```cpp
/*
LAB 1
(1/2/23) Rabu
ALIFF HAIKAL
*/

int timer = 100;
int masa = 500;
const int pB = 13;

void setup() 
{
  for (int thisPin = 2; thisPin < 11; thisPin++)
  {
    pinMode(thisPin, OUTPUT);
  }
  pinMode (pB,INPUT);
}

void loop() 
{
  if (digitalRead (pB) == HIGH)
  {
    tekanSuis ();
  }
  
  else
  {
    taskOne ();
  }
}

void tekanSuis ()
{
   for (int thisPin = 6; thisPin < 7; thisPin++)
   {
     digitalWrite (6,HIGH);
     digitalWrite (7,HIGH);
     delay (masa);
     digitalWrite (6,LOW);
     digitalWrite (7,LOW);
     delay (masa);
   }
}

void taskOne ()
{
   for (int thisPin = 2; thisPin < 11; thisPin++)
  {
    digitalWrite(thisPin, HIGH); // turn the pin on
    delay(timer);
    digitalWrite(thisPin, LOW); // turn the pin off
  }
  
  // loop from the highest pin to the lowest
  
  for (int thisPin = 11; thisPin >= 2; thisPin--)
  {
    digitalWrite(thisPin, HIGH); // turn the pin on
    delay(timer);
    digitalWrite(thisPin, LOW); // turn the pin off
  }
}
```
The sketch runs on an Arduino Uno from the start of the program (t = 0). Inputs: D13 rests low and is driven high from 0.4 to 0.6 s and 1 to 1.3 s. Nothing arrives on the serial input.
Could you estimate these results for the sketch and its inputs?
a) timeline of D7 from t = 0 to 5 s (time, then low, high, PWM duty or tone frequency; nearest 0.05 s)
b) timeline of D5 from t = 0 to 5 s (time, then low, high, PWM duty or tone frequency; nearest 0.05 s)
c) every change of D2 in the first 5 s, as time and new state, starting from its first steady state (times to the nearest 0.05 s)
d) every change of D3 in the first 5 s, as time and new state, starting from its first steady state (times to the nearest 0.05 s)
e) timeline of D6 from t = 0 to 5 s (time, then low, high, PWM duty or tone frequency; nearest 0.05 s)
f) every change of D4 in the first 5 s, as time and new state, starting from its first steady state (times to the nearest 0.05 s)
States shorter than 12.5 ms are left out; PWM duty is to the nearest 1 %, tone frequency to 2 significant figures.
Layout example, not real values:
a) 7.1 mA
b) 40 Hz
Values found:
a) 0 s low; 0.5 s high; 0.6 s low; 1.3 s high; 1.4 s low; 2.4 s high; 2.5 s low; 3.2 s high; 3.3 s low; 4.3 s high; 4.4 s low
b) 0 s low; 0.3 s high; 0.4 s low; 1.5 s high; 1.6 s low; 2.2 s high; 2.3 s low; 3.4 s high; 3.5 s low; 4.1 s high; 4.2 s low
c) 0 s high; 0.1 s low; 1.8 s high; 2 s low; 3.7 s high; 3.9 s low
d) 0 s low; 0.1 s high; 0.2 s low; 1.7 s high; 1.8 s low; 2 s high; 2.1 s low; 3.6 s high; 3.7 s low; 3.9 s high; 4 s low
e) 0 s low; 0.4 s high; 0.5 s low; 1.4 s high; 1.5 s low; 2.3 s high; 2.4 s low; 3.3 s high; 3.4 s low; 4.2 s high; 4.3 s low
f) 0 s low; 0.2 s high; 0.3 s low; 1.6 s high; 1.7 s low; 2.1 s high; 2.2 s low; 3.5 s high; 3.6 s low; 4 s high; 4.1 s low
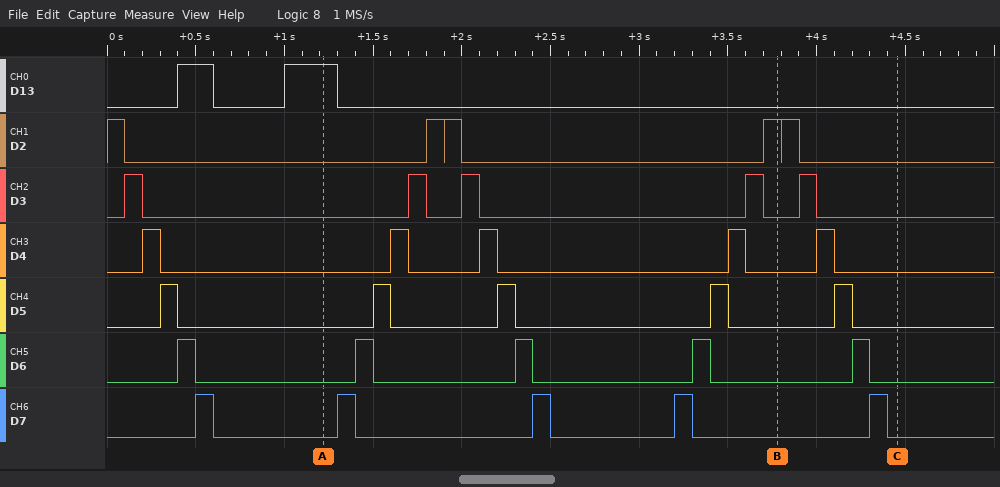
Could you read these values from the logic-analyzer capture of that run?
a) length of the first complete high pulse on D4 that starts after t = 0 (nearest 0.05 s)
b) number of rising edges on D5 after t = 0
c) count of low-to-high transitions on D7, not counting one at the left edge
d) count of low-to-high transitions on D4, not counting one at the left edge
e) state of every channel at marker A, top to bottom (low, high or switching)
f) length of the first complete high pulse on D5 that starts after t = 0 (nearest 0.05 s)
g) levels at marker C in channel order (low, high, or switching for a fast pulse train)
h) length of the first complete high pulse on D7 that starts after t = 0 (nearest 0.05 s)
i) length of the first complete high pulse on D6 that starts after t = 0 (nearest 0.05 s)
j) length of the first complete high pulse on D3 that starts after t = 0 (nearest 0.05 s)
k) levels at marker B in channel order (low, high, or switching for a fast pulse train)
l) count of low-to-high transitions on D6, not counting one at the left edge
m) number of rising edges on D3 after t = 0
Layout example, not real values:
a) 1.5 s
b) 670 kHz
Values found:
a) 0.10 s
b) 5
c) 5
d) 5
e) D13 high, D2 low, D3 low, D4 low, D5 low, D6 low, D7 low
f) 0.10 s
g) D13 low, D2 low, D3 low, D4 low, D5 low, D6 low, D7 low
h) 0.10 s
i) 0.10 s
j) 0.10 s
k) D13 low, D2 high, D3 low, D4 low, D5 low, D6 low, D7 low
l) 5
m) 5
